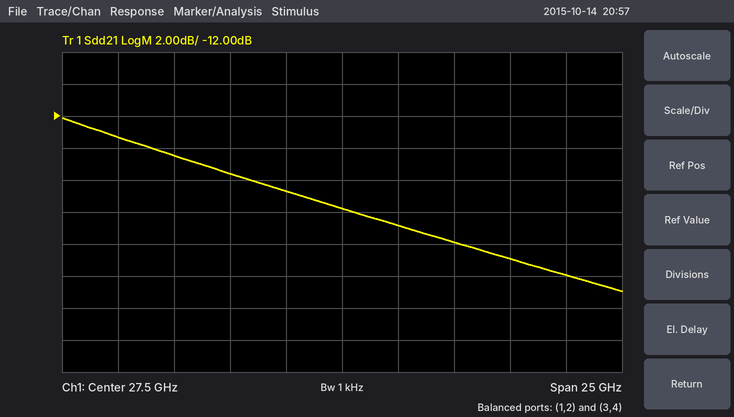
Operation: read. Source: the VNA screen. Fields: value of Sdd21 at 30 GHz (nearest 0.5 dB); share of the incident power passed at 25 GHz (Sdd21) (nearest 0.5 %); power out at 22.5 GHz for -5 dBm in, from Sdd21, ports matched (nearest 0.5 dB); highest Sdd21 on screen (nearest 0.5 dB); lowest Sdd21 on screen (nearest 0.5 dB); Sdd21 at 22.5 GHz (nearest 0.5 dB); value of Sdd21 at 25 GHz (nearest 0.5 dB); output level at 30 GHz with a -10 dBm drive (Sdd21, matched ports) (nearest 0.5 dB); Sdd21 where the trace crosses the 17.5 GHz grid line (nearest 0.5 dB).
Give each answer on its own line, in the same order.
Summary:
-19.0 dB
2.0 %
-20.5 dBm
-12.0 dB
-23.0 dB
-15.5 dB
-16.5 dB
-29.0 dBm
-13.5 dB
